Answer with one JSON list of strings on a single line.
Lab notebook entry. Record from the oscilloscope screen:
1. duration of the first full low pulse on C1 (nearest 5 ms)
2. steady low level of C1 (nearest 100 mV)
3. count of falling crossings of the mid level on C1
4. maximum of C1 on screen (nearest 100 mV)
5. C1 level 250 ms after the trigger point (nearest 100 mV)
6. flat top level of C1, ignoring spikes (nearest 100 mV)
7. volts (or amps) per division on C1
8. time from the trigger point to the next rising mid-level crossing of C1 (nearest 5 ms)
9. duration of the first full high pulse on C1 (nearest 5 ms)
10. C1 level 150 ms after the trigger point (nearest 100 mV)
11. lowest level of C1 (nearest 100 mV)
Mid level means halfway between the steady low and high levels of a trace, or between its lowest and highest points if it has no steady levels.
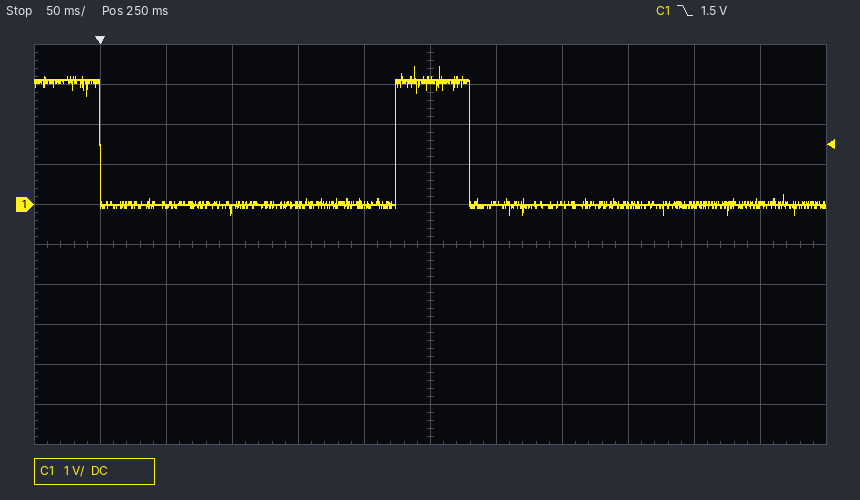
["225 ms", "0.0 V", "2", "3.4 V", "3.1 V", "3.1 V", "1 V", "225 ms", "55 ms", "0.0 V", "-200 mV"]
